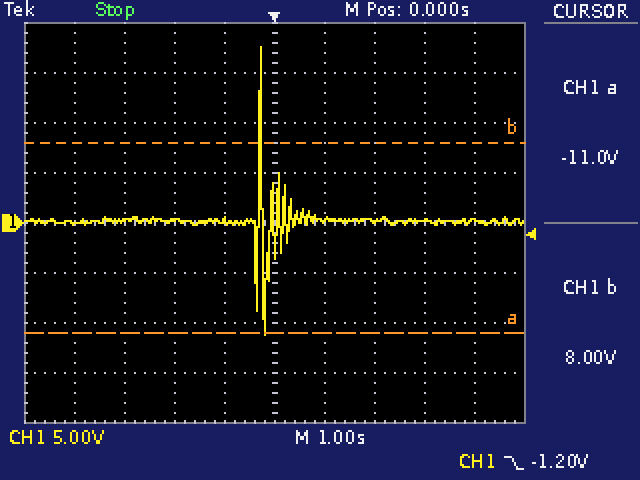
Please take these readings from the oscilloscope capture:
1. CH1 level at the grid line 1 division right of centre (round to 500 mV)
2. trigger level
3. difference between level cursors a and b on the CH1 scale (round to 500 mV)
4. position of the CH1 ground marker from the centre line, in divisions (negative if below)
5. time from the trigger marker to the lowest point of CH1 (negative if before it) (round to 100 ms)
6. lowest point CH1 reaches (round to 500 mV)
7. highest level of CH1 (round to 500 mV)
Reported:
500 mV
-1.20 V
19.0 V
0.0 div
-200 ms
-11.0 V
17.5 V
